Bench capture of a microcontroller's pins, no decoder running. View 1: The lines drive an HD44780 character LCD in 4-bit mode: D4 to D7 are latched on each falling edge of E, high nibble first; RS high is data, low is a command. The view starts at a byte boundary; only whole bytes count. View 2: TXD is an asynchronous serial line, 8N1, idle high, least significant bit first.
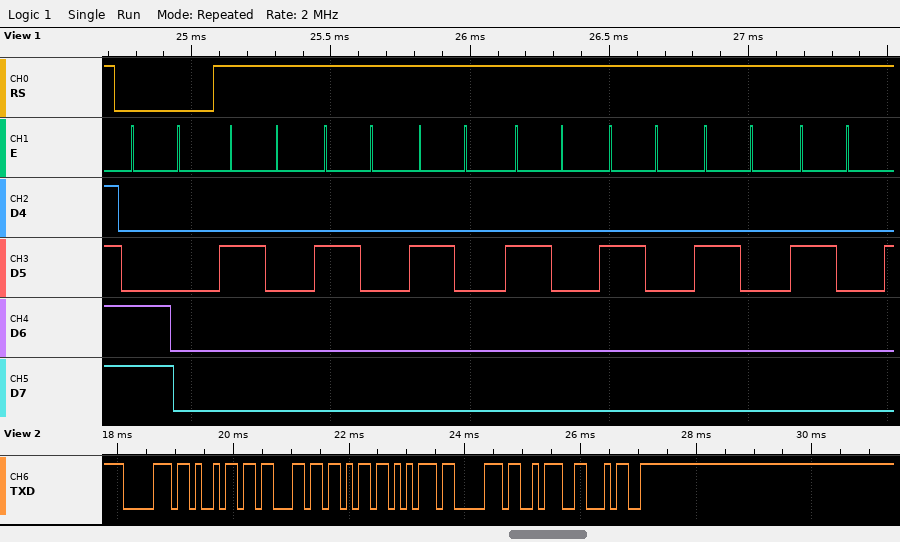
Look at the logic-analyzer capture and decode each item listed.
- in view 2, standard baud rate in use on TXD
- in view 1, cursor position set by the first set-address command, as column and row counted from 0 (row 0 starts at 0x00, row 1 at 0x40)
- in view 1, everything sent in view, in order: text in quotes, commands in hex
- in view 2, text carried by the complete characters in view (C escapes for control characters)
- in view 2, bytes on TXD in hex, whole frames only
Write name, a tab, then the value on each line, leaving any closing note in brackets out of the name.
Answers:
in view 2, standard baud rate in use on TXD	9600 baud
in view 1, cursor position set by the first set-address command, as column and row counted from 0	column 0, row 1
in view 1, everything sent in view, in order: text in quotes, commands in hex	0xC0 "       "
in view 2, text carried by the complete characters in view	"pickup:4"
in view 2, bytes on TXD in hex, whole frames only	0x70 0x69 0x63 0x6B 0x75 0x70 0x3A 0x34
